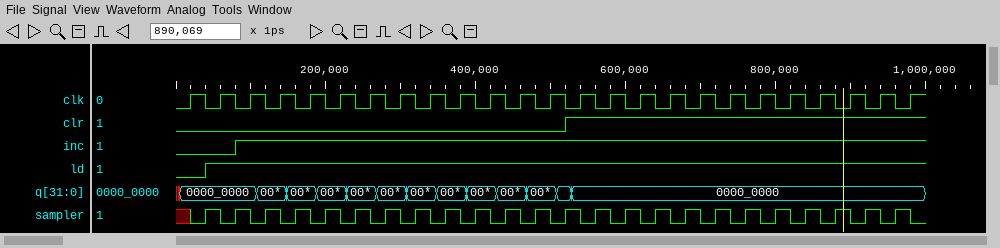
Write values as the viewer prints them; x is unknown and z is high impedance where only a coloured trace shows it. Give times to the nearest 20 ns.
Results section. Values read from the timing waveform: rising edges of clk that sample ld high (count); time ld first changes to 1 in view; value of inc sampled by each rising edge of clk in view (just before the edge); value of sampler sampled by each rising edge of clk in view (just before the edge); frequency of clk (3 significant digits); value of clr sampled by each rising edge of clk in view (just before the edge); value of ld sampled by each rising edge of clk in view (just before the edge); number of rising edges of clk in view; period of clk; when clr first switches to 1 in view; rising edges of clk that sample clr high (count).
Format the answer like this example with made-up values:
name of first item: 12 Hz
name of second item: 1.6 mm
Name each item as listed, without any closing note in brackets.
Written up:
rising edges of clk that sample ld high: 24
time ld first changes to 1 in view: 40 ns
value of inc sampled by each rising edge of clk in view: 0 0 1 1 1 1 1 1 1 1 1 1 1 1 1 1 1 1 1 1 1 1 1 1 1
value of sampler sampled by each rising edge of clk in view: x 1 1 1 1 1 1 1 1 1 1 1 1 1 1 1 1 1 1 1 1 1 1 1 1
frequency of clk: 25.0 MHz
value of clr sampled by each rising edge of clk in view: 0 0 0 0 0 0 0 0 0 0 0 0 0 1 1 1 1 1 1 1 1 1 1 1 1
value of ld sampled by each rising edge of clk in view: 0 1 1 1 1 1 1 1 1 1 1 1 1 1 1 1 1 1 1 1 1 1 1 1 1
number of rising edges of clk in view: 25
period of clk: 40 ns
when clr first switches to 1 in view: 520 ns
rising edges of clk that sample clr high: 12
